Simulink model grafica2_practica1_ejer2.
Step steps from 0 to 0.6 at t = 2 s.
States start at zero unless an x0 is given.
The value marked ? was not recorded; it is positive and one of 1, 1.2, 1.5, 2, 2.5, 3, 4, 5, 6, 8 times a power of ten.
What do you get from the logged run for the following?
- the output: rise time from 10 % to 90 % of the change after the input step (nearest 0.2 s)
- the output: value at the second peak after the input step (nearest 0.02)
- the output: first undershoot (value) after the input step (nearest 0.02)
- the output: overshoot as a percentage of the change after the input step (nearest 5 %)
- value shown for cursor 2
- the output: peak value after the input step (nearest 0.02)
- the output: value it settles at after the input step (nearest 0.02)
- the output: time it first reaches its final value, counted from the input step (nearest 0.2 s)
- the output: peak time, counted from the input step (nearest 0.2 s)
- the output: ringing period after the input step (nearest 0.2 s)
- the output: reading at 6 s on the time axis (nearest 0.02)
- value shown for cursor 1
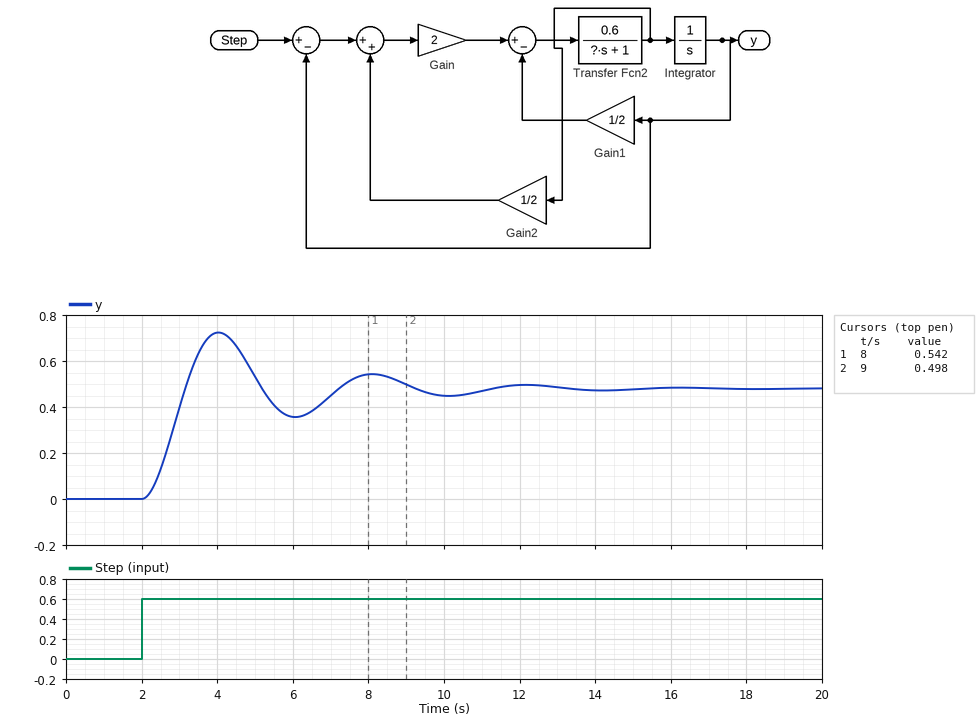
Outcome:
0.8 s
0.54
0.36
50 %
0.498
0.72
0.48
1.2 s
2.0 s
4.0 s
0.36
0.542
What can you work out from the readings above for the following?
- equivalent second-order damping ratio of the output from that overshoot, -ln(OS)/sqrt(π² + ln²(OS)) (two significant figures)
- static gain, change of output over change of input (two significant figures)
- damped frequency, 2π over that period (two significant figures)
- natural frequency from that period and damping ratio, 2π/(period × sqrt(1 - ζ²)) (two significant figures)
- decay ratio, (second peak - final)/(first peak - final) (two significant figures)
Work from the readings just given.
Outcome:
0.22
0.80
1.6 rad/s
1.6 rad/s
0.25
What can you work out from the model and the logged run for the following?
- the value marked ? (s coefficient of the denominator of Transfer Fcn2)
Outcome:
0.6
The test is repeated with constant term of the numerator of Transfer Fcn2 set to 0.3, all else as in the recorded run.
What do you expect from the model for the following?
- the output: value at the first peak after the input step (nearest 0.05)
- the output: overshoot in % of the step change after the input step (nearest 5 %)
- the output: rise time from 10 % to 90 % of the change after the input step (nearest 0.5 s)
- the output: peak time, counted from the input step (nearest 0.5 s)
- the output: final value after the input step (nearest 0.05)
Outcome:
0.55
15 %
1.5 s
3.5 s
0.50
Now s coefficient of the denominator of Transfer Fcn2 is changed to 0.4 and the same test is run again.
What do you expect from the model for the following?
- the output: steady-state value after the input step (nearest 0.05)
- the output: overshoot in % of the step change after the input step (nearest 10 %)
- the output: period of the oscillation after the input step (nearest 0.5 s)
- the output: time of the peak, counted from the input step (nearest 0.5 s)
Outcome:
0.50
40 %
3.5 s
1.5 s
